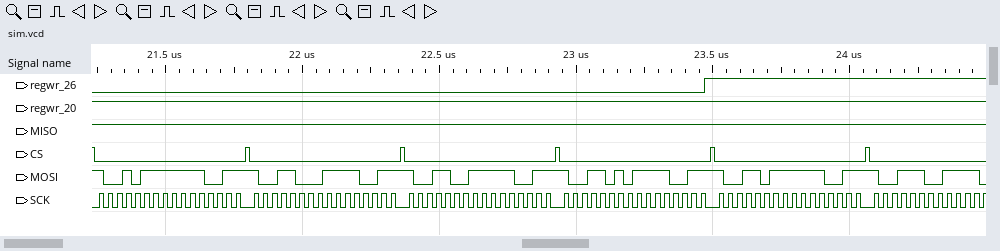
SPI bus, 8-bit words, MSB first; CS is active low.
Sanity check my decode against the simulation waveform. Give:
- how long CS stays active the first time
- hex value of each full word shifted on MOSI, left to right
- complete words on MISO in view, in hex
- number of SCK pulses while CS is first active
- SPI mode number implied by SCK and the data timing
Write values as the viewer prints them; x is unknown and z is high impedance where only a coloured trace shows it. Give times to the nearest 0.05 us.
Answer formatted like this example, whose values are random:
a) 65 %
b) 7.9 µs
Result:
a) 0.55 us
b) 97, F3, 98, F3, 99, F3, 9A, F3, 9B, F3, 9C
c) FF, FF, FF, FF, FF, FF, FF, FF, FF, FF, FF
d) 16
e) 0
